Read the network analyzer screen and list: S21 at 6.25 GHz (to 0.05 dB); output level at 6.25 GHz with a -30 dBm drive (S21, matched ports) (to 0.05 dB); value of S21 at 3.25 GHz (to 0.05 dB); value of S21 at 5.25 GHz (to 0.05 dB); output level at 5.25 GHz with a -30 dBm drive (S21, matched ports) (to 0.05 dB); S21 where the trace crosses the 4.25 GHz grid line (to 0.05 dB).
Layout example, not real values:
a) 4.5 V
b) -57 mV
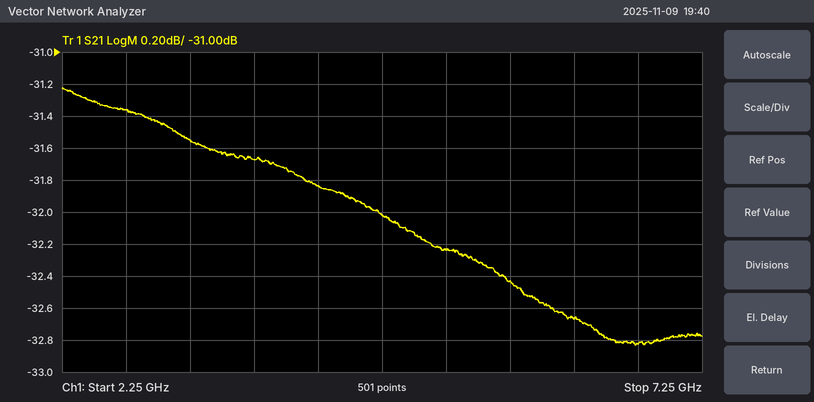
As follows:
a) -32.65 dB
b) -62.65 dBm
c) -31.55 dB
d) -32.25 dB
e) -62.25 dBm
f) -31.85 dB
